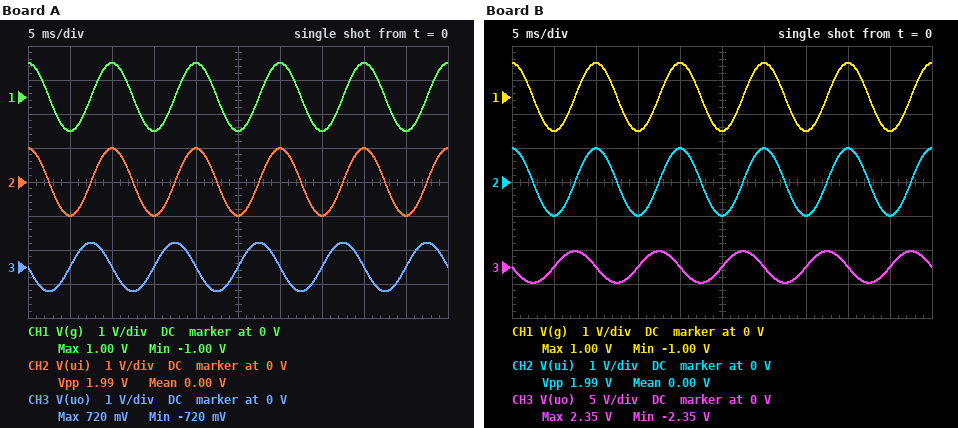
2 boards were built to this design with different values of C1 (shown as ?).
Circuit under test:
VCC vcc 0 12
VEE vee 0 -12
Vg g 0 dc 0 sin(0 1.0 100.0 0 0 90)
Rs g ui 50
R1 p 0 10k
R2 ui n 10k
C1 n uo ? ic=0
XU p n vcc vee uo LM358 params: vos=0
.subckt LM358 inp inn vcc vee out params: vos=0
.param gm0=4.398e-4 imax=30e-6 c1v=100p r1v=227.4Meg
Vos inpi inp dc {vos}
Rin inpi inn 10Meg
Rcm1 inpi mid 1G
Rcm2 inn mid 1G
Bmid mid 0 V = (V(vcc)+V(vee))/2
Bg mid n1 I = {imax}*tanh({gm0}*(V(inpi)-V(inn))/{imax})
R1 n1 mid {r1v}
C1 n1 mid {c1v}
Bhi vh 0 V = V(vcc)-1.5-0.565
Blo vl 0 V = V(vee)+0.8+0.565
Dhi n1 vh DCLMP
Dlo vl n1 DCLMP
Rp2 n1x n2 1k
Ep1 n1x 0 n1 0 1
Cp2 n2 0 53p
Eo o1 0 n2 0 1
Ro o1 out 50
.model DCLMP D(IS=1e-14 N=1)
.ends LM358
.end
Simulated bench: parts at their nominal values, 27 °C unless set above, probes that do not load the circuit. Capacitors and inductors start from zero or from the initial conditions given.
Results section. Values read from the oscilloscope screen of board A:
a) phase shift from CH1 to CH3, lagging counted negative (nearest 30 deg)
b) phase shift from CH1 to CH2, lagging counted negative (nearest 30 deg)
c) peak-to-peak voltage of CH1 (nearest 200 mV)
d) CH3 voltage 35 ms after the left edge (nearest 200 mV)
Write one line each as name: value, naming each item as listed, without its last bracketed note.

phase shift from CH1 to CH3, lagging counted negative: 90 deg
phase shift from CH1 to CH2, lagging counted negative: 0 deg
peak-to-peak voltage of CH1: 2.0 V
CH3 voltage 35 ms after the left edge: 0 V
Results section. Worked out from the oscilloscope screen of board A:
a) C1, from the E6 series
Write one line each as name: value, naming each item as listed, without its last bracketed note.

C1, from the E6 series: 220 nF
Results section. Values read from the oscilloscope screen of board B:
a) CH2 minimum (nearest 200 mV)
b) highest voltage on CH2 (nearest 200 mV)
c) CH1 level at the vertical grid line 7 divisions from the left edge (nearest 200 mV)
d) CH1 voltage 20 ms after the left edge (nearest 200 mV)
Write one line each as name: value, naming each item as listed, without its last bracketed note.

CH2 minimum: -1.0 V
highest voltage on CH2: 1.0 V
CH1 level at the vertical grid line 7 divisions from the left edge: -1.0 V
CH1 voltage 20 ms after the left edge: 1.0 V
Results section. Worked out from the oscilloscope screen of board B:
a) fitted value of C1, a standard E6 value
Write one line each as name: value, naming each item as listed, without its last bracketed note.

fitted value of C1, a standard E6 value: 68 nF
